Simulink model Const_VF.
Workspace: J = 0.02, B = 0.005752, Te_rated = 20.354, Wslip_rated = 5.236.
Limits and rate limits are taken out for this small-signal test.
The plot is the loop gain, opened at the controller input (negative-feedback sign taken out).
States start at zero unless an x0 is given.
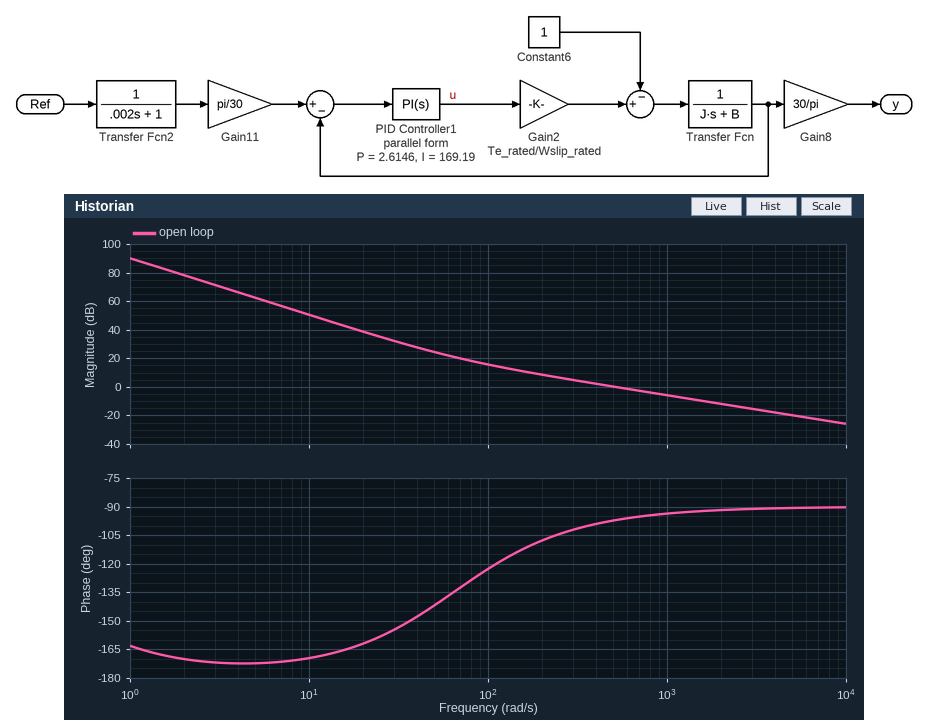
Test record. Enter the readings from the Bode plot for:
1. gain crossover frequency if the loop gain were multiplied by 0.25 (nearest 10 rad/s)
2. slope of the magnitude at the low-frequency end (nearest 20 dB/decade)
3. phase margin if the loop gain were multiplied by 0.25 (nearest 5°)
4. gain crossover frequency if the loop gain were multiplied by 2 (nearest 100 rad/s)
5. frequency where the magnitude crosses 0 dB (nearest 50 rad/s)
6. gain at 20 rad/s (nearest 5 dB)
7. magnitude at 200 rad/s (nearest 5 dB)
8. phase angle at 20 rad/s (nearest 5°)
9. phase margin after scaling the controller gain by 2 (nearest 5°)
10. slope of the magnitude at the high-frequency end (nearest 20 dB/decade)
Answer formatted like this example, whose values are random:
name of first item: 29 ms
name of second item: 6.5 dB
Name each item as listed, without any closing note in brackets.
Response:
gain crossover frequency if the loop gain were multiplied by 0.25: 140 rad/s
slope of the magnitude at the low-frequency end: -40 dB/decade
phase margin if the loop gain were multiplied by 0.25: 65°
gain crossover frequency if the loop gain were multiplied by 2: 1000 rad/s
frequency where the magnitude crosses 0 dB: 500 rad/s
gain at 20 rad/s: 40 dB
magnitude at 200 rad/s: 10 dB
phase angle at 20 rad/s: -160°
phase margin after scaling the controller gain by 2: 85°
slope of the magnitude at the high-frequency end: -20 dB/decade
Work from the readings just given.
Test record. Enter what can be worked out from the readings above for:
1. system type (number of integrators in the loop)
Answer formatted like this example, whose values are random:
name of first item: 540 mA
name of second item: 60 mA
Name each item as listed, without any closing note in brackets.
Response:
system type: 2
